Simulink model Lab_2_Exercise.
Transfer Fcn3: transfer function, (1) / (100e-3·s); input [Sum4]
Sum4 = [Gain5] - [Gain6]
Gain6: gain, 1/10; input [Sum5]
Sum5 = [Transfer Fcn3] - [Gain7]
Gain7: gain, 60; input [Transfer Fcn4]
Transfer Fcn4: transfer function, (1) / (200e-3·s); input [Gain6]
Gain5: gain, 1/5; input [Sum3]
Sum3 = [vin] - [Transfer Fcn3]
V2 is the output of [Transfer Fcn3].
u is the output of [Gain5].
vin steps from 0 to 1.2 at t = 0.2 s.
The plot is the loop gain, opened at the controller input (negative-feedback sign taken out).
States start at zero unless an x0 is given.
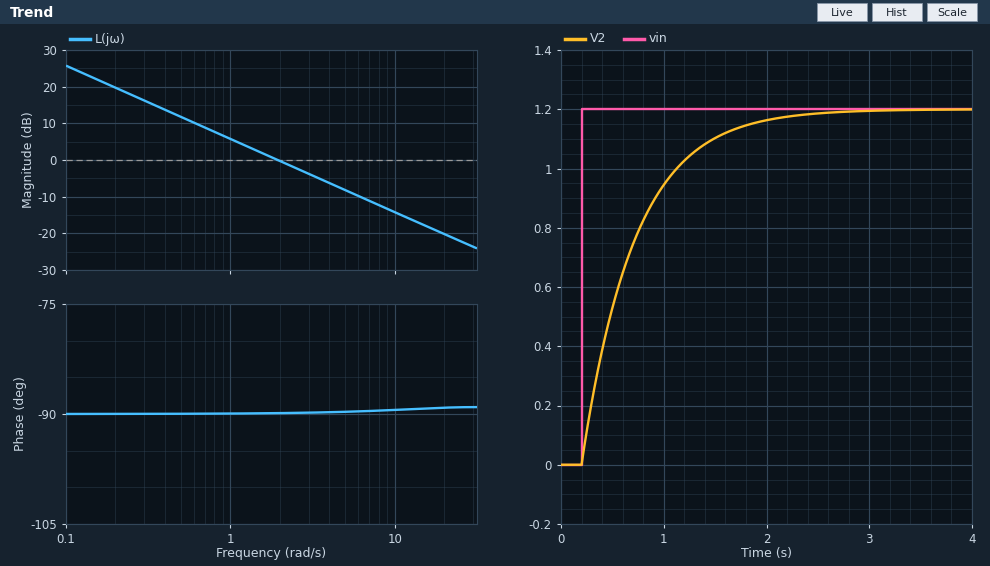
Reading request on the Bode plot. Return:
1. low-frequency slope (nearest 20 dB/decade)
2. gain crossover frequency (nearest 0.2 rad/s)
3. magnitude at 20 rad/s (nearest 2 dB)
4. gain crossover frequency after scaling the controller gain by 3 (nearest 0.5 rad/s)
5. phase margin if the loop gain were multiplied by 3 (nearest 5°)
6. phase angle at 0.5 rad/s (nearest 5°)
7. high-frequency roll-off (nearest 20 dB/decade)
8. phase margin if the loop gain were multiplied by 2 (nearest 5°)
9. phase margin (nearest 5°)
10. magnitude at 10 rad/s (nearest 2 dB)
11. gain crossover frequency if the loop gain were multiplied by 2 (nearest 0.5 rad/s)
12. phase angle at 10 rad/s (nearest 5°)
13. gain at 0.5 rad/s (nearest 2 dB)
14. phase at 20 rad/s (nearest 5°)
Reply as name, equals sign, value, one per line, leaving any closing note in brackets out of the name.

low-frequency slope = -20 dB/decade
gain crossover frequency = 2.0 rad/s
magnitude at 20 rad/s = -20 dB
gain crossover frequency after scaling the controller gain by 3 = 6.0 rad/s
phase margin if the loop gain were multiplied by 3 = 90°
phase angle at 0.5 rad/s = -90°
high-frequency roll-off = -20 dB/decade
phase margin if the loop gain were multiplied by 2 = 90°
phase margin = 90°
magnitude at 10 rad/s = -14 dB
gain crossover frequency if the loop gain were multiplied by 2 = 4.0 rad/s
phase angle at 10 rad/s = -90°
gain at 0.5 rad/s = 12 dB
phase at 20 rad/s = -90°
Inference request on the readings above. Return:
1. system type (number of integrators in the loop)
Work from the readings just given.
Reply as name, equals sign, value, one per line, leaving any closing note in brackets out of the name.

system type = 1
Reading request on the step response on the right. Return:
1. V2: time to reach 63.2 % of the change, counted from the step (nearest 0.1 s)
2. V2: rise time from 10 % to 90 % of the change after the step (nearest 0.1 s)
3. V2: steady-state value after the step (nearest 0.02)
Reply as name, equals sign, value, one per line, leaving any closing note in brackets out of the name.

V2: time to reach 63.2 % of the change, counted from the step = 0.5 s
V2: rise time from 10 % to 90 % of the change after the step = 1.1 s
V2: steady-state value after the step = 1.20
